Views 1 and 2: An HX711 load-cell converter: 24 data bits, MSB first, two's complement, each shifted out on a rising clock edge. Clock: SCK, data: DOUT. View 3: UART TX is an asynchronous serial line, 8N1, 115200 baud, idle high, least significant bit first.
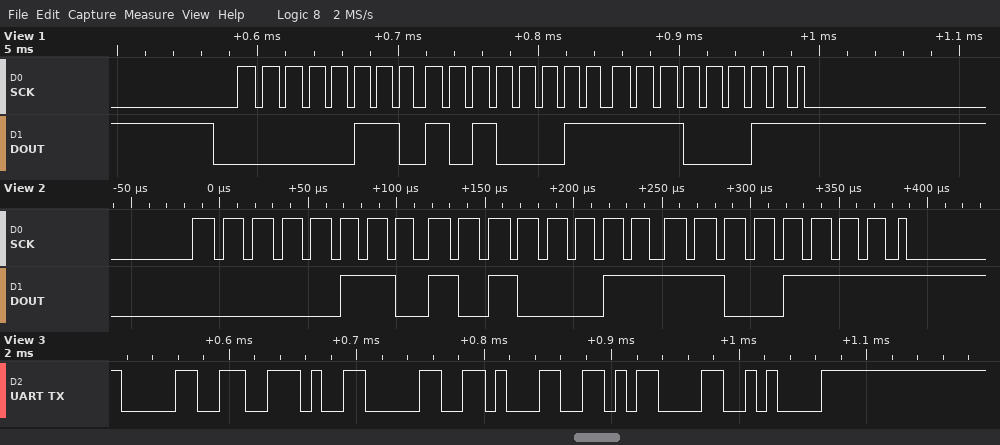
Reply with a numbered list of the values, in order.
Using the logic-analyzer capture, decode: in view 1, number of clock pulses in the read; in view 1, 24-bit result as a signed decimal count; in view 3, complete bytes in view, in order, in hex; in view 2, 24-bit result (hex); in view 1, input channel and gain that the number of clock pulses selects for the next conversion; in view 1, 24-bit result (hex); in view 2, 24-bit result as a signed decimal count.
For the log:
1. 25
2. 435171
3. 30 2E 30 31 0D 0A
4. 0x06A3CF
5. channel A, gain 128
6. 0x06A3E3
7. 435151
